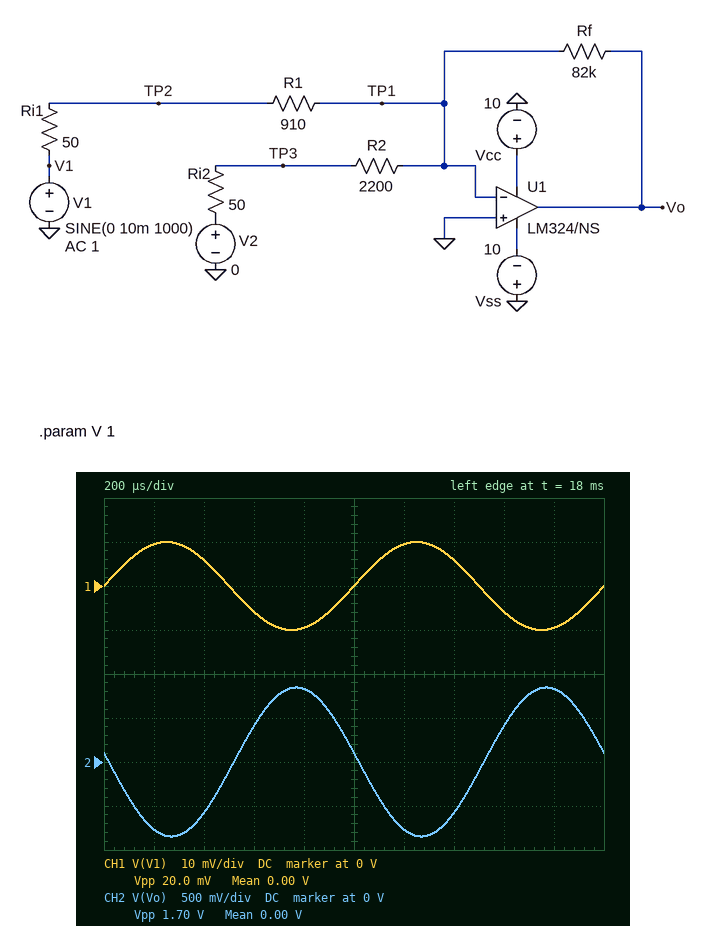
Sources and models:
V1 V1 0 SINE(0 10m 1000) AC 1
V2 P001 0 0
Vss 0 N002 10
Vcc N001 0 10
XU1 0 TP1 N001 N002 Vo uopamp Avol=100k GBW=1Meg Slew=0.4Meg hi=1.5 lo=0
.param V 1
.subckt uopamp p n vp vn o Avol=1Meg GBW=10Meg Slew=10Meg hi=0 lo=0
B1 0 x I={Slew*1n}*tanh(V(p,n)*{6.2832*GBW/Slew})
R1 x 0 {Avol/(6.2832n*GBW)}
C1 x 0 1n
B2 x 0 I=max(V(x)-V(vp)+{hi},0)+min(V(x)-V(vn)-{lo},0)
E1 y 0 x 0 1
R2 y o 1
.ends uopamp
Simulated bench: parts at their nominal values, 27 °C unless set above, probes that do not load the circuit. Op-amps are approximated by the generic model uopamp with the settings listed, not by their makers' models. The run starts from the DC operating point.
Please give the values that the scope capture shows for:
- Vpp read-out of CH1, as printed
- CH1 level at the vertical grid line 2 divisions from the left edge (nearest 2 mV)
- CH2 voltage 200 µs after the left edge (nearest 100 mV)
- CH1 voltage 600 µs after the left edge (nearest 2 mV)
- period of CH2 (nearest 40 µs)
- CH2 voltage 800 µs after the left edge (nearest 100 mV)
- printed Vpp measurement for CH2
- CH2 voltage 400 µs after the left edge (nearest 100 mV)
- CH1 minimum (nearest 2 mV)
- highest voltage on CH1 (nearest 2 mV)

20.0 mV
6 mV
-800 mV
-6 mV
1.00 ms
800 mV
1.70 V
-600 mV
-10 mV
10 mV
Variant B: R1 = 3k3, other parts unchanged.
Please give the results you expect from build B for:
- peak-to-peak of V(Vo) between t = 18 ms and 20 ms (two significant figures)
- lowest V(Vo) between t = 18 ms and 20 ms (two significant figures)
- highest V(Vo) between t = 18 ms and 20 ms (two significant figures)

490 mV
-240 mV
240 mV
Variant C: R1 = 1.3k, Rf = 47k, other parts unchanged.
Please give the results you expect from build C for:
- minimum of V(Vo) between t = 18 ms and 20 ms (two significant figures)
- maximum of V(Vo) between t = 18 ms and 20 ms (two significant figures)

-350 mV
350 mV
